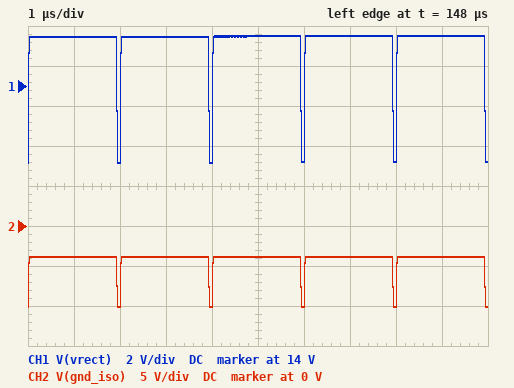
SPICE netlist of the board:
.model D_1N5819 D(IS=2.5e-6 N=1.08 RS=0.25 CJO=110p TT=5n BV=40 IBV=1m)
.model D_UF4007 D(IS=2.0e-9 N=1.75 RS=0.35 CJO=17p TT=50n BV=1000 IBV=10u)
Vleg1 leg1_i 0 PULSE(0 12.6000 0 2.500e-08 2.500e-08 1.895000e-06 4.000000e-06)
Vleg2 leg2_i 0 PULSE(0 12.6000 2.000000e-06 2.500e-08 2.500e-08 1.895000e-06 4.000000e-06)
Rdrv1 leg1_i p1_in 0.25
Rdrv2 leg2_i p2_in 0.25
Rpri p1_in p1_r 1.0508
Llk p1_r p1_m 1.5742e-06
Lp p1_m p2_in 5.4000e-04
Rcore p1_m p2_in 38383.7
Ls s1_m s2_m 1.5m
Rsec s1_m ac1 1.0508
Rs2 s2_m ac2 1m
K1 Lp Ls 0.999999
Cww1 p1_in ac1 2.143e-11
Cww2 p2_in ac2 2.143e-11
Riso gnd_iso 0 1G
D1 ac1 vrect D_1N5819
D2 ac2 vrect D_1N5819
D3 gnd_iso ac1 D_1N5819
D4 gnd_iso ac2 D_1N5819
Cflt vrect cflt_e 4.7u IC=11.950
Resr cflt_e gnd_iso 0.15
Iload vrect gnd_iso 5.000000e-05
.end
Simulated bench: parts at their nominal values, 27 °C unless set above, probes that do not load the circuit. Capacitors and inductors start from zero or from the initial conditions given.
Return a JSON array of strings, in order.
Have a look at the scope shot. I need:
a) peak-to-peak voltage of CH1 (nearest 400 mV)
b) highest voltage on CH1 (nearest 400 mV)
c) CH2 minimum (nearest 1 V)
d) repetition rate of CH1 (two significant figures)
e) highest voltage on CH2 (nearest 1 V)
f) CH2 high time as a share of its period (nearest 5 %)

["6.4 V", "16.4 V", "-10 V", "500 kHz", "-4 V", "95 %"]
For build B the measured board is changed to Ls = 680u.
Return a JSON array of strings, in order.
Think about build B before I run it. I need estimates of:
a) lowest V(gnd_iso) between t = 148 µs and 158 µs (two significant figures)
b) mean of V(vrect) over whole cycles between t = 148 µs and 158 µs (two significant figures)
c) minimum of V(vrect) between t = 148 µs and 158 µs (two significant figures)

["-6.9 V", "13 V", "6.9 V"]
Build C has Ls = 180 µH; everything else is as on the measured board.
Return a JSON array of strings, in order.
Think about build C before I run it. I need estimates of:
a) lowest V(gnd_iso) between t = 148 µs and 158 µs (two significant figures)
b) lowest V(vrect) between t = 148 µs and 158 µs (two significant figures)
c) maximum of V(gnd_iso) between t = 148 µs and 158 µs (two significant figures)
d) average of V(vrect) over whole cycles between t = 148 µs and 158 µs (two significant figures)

["-6.0 V", "6.0 V", "330 mV", "12 V"]
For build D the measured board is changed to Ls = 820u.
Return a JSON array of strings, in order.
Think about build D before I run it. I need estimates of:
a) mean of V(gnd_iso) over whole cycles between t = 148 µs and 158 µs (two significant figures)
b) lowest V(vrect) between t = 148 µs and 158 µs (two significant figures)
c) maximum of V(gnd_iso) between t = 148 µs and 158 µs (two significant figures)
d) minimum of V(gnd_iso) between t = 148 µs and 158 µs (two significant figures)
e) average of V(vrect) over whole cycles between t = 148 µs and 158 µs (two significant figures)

["-1.5 V", "7.6 V", "-1.3 V", "-7.6 V", "14 V"]
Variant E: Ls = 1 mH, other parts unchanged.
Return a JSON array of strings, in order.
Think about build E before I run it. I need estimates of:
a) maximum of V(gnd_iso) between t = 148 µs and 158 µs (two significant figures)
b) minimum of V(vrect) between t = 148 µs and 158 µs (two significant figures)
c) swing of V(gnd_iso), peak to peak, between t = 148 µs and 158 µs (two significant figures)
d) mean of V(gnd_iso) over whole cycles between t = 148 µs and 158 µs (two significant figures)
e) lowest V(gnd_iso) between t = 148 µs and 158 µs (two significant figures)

["-2.1 V", "8.4 V", "6.3 V", "-2.3 V", "-8.4 V"]
